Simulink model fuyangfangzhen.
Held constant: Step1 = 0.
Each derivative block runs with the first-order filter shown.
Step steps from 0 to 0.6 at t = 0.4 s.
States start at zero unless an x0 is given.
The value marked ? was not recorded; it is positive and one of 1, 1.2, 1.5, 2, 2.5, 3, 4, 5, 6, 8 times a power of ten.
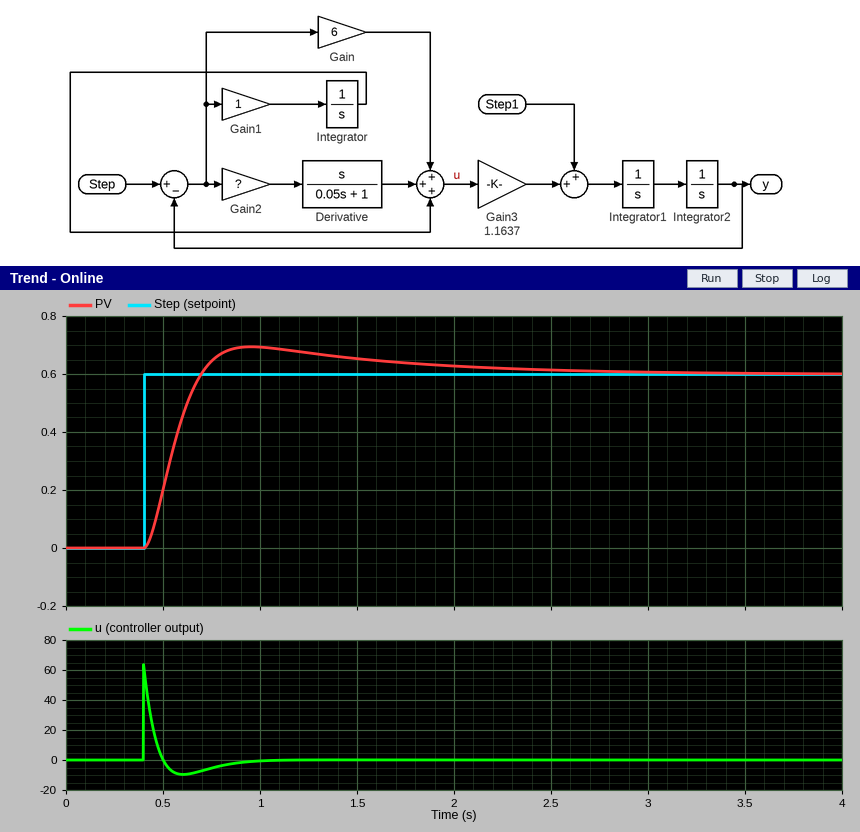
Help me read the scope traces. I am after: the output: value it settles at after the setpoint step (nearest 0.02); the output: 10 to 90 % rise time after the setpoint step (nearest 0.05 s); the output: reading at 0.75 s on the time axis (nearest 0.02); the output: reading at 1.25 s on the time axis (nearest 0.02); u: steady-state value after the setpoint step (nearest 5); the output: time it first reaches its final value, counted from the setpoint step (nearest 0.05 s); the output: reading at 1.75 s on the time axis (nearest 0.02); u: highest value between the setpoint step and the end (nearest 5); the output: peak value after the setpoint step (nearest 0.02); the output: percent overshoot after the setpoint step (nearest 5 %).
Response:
0.60
0.20 s
0.64
0.68
0
0.30 s
0.64
65
0.70
15 %
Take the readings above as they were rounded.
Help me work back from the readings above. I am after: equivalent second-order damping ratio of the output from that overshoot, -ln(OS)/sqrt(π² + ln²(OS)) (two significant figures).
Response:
0.52
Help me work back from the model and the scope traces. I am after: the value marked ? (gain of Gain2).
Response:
5
